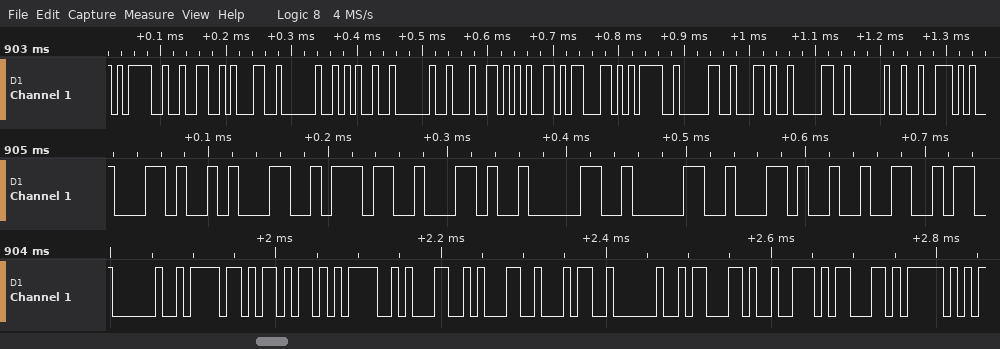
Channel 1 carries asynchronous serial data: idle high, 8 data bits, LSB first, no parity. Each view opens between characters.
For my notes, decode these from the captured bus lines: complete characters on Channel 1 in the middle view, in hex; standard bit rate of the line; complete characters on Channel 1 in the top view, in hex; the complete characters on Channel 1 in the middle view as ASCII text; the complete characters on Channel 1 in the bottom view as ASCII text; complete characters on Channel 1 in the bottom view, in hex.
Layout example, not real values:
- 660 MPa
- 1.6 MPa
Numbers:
- 2C, 31, 37, 2C, 30, 30, 2C, 32
- 115200 baud
- 3D, 32, 31, 20, 25, 20, 64, 65, 63, 3D, 30, 2C, 30, 20, 72
- ",17,00,2"
- " ok=114 crc_"
- 20, 6F, 6B, 3D, 31, 31, 34, 20, 63, 72, 63, 5F
